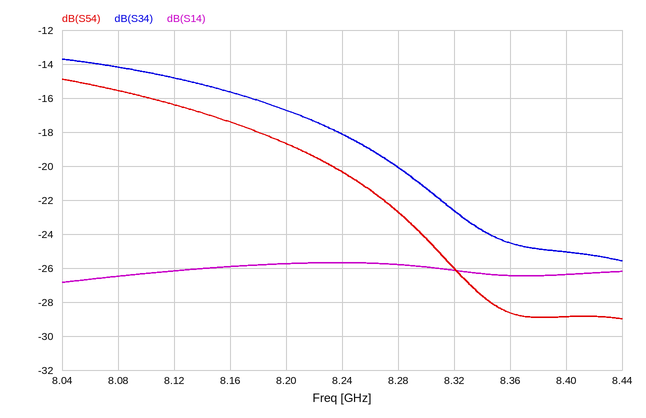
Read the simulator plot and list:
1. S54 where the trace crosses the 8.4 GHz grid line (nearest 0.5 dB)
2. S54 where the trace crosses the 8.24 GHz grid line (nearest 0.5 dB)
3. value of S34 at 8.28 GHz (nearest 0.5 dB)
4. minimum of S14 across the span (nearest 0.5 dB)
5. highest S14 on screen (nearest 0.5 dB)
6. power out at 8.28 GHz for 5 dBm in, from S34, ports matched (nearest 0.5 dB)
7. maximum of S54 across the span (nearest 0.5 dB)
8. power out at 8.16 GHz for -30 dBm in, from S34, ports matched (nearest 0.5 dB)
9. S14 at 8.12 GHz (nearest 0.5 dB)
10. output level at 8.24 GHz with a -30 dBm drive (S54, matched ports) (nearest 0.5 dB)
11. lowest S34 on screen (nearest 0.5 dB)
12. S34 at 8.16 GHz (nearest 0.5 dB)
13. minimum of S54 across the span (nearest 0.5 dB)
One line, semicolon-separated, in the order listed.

-29.0 dB; -20.5 dB; -20.0 dB; -27.0 dB; -25.5 dB; -15.0 dBm; -15.0 dB; -45.5 dBm; -26.0 dB; -50.5 dBm; -25.5 dB; -15.5 dB; -29.0 dB
